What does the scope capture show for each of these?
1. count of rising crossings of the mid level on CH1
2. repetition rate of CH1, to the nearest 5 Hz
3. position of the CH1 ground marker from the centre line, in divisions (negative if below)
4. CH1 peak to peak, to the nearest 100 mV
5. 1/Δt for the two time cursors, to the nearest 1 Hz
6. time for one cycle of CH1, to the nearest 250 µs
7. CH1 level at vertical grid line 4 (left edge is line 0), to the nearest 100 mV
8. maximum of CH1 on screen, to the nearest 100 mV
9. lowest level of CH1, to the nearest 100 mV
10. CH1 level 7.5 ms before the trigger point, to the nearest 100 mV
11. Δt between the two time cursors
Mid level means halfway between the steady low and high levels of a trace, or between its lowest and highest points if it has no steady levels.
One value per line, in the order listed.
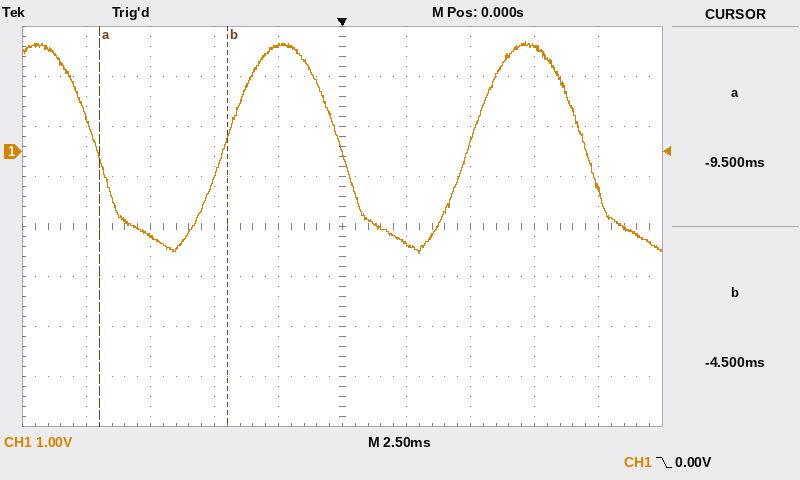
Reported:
2
105 Hz
+1.5 div
4.2 V
200 Hz
9.50 ms
2.1 V
2.2 V
-2.0 V
-1.7 V
5.00 ms
